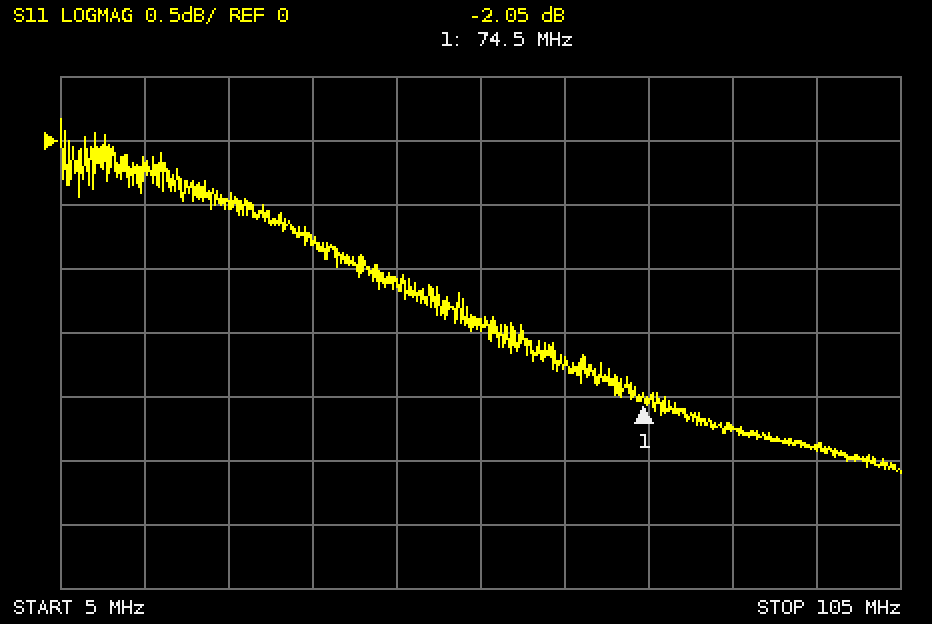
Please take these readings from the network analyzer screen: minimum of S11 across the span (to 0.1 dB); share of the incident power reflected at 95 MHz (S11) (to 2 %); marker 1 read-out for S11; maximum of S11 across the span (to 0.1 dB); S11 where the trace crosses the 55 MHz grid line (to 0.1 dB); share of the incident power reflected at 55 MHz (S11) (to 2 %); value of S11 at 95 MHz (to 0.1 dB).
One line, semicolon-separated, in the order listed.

-2.6 dB; 58 %; -2.05 dB; 0.2 dB; -1.4 dB; 72 %; -2.4 dB
